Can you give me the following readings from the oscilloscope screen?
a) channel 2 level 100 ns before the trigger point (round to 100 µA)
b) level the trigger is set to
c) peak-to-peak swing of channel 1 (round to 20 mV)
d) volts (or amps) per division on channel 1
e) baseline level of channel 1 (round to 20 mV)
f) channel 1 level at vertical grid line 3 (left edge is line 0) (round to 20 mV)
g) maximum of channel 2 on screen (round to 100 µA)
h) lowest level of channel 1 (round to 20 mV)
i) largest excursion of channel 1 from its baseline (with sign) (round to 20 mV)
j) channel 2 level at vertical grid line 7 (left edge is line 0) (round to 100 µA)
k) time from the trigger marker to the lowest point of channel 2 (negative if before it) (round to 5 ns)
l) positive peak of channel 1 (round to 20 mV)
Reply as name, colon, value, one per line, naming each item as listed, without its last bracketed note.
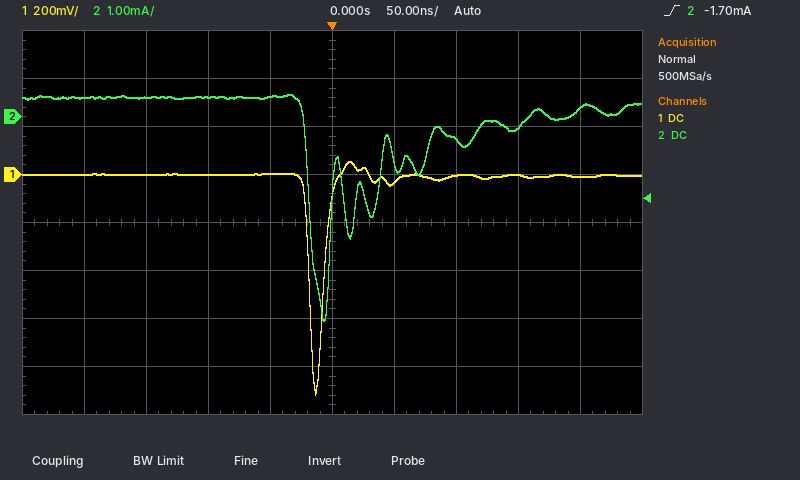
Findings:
channel 2 level 100 ns before the trigger point: 400 µA
level the trigger is set to: -1.70 mA
peak-to-peak swing of channel 1: 980 mV
volts (or amps) per division on channel 1: 200 mV
baseline level of channel 1: 0 mV
channel 1 level at vertical grid line 3 (left edge is line 0): 0 mV
maximum of channel 2 on screen: 500 µA
lowest level of channel 1: -920 mV
largest excursion of channel 1 from its baseline (with sign): -920 mV
channel 2 level at vertical grid line 7 (left edge is line 0): -500 µA
time from the trigger marker to the lowest point of channel 2 (negative if before it): -5 ns
positive peak of channel 1: 60 mV
